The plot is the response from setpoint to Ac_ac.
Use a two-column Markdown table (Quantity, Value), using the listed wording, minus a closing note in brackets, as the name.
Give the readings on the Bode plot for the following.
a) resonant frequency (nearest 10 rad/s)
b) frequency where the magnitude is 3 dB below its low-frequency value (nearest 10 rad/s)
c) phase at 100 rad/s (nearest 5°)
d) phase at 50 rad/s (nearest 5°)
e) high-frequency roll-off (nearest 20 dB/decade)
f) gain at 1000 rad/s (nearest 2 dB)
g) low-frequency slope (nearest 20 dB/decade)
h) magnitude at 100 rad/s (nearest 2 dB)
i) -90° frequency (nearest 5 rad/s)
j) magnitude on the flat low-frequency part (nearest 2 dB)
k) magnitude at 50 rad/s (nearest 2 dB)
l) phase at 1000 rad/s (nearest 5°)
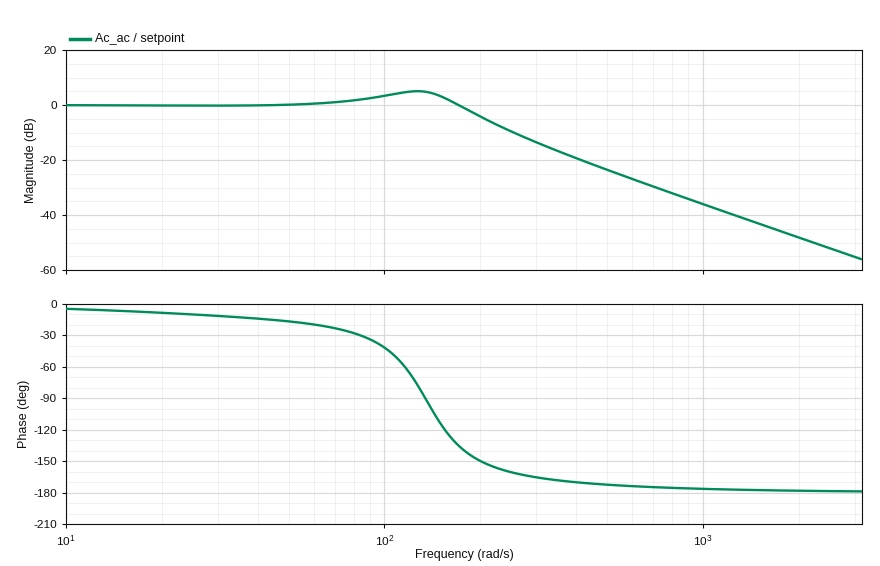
| Quantity | Value |
|---|---|
| resonant frequency | 130 rad/s |
| frequency where the magnitude is 3 dB below its low-frequency value | 190 rad/s |
| phase at 100 rad/s | -40° |
| phase at 50 rad/s | -15° |
| high-frequency roll-off | -40 dB/decade |
| gain at 1000 rad/s | -36 dB |
| low-frequency slope | 0 dB/decade |
| magnitude at 100 rad/s | 4 dB |
| -90° frequency | 135 rad/s |
| magnitude on the flat low-frequency part | 0 dB |
| magnitude at 50 rad/s | 0 dB |
| phase at 1000 rad/s | -175° |
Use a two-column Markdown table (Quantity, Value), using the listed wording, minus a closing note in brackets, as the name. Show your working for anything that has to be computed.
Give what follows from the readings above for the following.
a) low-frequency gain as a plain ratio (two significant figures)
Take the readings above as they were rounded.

| Quantity | Value |
|---|---|
| low-frequency gain as a plain ratio | 10^(0 / 20) = 1.0 |
